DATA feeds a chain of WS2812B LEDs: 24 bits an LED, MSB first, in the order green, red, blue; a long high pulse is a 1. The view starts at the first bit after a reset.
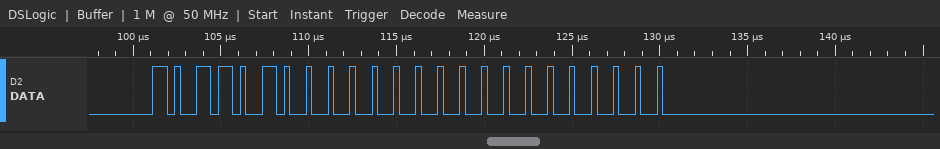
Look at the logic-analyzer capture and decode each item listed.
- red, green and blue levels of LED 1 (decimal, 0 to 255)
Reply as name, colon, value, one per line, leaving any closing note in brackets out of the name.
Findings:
red, green and blue levels of LED 1: 0, 180, 0
